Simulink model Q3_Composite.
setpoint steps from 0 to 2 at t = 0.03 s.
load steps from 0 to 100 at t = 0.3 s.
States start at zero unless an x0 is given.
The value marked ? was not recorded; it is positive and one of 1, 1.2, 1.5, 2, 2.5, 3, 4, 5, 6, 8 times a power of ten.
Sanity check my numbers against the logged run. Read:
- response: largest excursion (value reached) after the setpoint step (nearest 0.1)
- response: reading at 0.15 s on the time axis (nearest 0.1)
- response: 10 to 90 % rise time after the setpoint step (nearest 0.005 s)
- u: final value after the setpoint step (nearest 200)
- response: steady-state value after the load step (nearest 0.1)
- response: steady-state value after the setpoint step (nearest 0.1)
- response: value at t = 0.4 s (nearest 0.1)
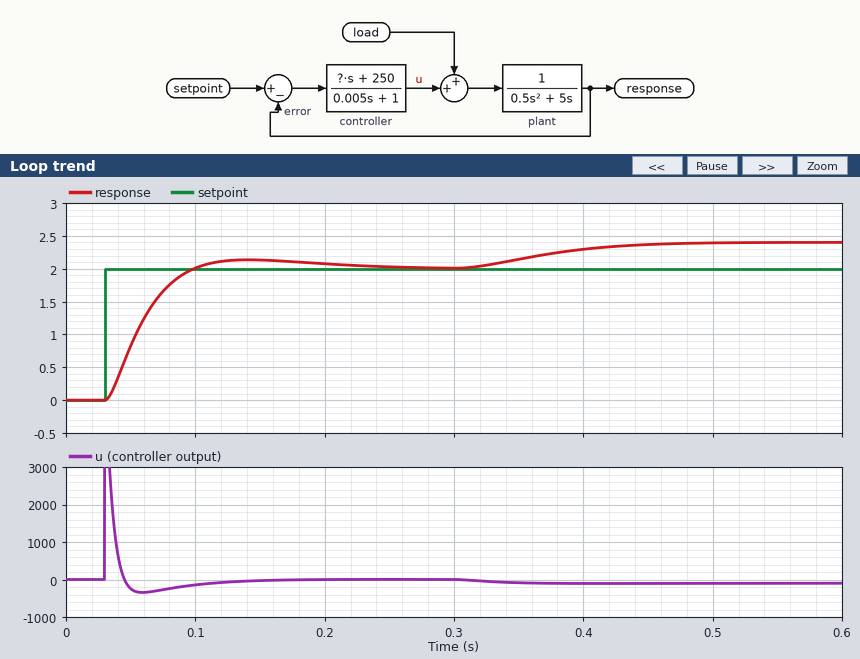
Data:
2.1
2.1
0.045 s
0
2.4
2.0
2.3
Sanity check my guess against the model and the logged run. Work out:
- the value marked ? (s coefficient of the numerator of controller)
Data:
15
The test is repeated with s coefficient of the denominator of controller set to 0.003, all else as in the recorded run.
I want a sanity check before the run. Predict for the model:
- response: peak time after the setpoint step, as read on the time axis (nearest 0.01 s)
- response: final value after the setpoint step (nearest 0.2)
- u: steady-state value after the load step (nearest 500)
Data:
0.15 s
2.0
0
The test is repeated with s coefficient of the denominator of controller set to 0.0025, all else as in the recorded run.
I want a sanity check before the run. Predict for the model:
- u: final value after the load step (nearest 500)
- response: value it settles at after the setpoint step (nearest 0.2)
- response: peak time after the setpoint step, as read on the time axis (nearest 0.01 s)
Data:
0
2.0
0.15 s
